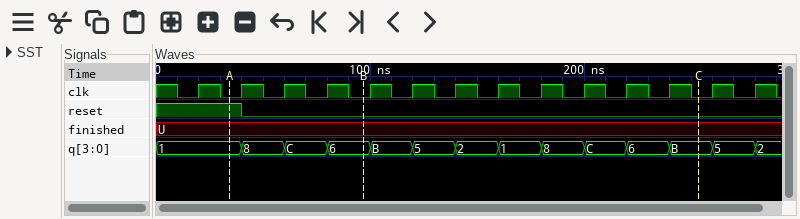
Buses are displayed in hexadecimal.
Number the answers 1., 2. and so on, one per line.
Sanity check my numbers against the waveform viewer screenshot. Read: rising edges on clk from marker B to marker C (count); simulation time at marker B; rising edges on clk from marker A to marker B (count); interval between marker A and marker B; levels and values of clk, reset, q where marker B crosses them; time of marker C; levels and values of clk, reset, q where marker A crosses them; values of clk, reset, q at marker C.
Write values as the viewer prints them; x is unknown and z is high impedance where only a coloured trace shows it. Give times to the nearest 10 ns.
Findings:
1. 8
2. 100 ns
3. 3
4. 60 ns
5. clk=0, reset=0, q=6
6. 250 ns
7. clk=0, reset=1, q=1
8. clk=0, reset=0, q=B
